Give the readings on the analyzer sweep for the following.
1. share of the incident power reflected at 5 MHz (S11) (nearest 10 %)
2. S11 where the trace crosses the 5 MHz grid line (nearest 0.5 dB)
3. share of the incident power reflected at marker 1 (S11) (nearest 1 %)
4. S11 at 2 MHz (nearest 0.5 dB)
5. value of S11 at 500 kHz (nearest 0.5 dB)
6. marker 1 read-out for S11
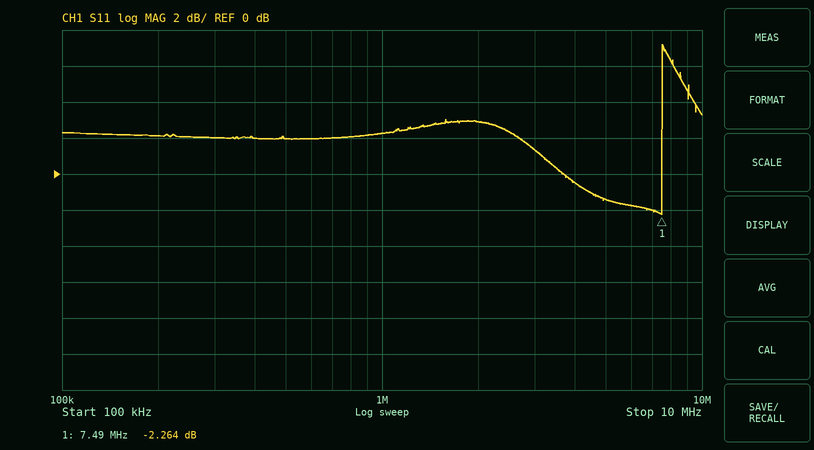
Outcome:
70 %
-1.5 dB
59 %
3.0 dB
2.0 dB
-2.264 dB
